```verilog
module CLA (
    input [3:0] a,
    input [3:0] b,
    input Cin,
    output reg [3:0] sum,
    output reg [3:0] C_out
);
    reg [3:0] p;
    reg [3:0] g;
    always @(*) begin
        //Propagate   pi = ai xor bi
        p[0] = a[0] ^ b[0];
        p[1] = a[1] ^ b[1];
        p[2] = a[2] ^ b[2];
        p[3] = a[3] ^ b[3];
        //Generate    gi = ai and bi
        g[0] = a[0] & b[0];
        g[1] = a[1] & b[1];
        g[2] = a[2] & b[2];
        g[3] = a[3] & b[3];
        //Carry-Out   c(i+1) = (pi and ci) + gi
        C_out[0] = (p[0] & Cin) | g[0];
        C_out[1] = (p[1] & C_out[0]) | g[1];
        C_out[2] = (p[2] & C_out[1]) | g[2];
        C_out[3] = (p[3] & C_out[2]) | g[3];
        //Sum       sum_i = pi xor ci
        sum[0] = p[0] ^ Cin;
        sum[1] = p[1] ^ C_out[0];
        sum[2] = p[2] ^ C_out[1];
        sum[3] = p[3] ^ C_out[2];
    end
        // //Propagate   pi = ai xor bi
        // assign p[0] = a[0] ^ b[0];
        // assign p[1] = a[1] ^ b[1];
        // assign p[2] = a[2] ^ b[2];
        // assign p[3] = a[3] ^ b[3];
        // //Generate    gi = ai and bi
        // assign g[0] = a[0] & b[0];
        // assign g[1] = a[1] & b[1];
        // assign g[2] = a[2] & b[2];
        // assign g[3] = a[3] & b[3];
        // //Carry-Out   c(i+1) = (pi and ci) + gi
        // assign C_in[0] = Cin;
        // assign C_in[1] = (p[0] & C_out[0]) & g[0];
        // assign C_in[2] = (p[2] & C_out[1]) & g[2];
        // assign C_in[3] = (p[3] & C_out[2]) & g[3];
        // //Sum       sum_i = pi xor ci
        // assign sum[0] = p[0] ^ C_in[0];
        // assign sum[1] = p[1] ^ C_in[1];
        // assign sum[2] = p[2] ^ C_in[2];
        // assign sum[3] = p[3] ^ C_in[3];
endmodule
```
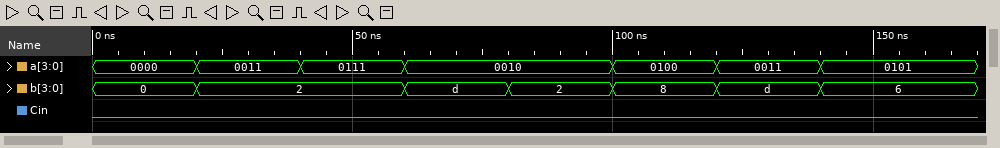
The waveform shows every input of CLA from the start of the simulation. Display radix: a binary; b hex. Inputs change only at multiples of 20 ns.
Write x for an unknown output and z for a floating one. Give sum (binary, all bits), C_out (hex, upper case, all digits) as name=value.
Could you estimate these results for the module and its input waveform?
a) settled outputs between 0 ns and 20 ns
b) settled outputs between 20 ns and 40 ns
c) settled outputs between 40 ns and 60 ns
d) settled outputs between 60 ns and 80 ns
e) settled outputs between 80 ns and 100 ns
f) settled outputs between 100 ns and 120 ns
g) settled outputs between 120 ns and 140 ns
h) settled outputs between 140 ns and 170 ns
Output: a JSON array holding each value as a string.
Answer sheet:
["sum=0000, C_out=0", "sum=0101, C_out=2", "sum=1001, C_out=6", "sum=1111, C_out=0", "sum=0100, C_out=2", "sum=1100, C_out=0", "sum=0000, C_out=F", "sum=1011, C_out=4"]
